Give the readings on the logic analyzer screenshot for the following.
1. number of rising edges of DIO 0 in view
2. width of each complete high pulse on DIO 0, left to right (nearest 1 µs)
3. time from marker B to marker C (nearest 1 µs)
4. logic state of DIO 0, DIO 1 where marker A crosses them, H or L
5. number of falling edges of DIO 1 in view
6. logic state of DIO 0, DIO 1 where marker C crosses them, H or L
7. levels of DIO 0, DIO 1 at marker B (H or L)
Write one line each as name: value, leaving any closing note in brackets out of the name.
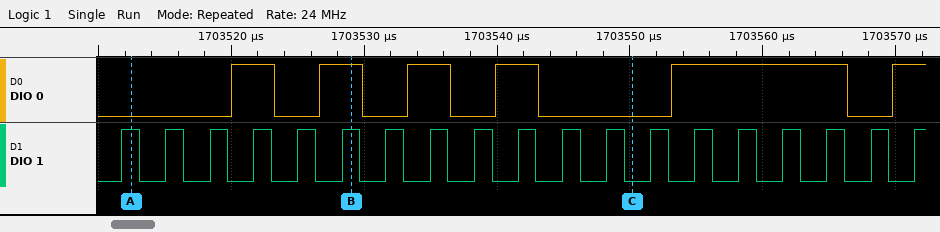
number of rising edges of DIO 0 in view: 6
width of each complete high pulse on DIO 0, left to right: 3 µs, 3 µs, 3 µs, 3 µs, 13 µs
time from marker B to marker C: 21 µs
logic state of DIO 0, DIO 1 where marker A crosses them, H or L: DIO 0=L, DIO 1=H
number of falling edges of DIO 1 in view: 18
logic state of DIO 0, DIO 1 where marker C crosses them, H or L: DIO 0=L, DIO 1=L
levels of DIO 0, DIO 1 at marker B: DIO 0=H, DIO 1=H
